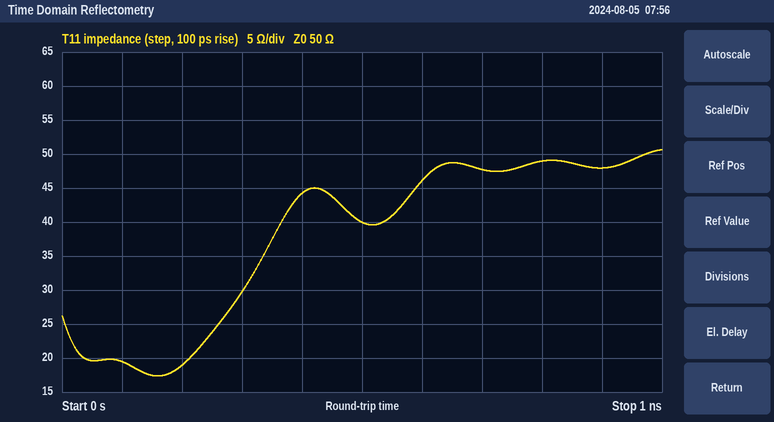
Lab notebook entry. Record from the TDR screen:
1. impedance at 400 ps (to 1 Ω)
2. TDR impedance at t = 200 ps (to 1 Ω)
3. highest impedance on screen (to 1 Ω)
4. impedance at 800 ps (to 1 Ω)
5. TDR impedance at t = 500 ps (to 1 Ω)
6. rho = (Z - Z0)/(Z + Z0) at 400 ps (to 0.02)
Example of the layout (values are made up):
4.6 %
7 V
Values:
44 Ω
19 Ω
51 Ω
49 Ω
40 Ω
-0.06
